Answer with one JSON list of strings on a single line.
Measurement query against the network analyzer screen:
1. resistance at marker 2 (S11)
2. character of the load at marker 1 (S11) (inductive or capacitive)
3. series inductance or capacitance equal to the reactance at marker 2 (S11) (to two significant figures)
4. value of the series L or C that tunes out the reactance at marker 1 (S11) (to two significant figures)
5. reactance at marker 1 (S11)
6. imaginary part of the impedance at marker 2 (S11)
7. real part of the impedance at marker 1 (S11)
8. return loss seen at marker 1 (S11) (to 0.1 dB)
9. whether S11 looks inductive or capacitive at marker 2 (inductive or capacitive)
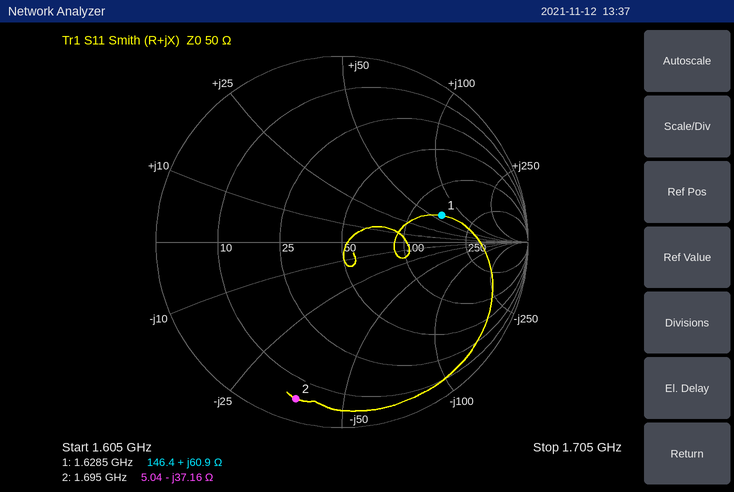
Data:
["5.04 Ω", "inductive", "2.5 pF", "1.6 pF", "+60.9 Ω", "-37.16 Ω", "146.4 Ω", "5.1 dB", "capacitive"]
